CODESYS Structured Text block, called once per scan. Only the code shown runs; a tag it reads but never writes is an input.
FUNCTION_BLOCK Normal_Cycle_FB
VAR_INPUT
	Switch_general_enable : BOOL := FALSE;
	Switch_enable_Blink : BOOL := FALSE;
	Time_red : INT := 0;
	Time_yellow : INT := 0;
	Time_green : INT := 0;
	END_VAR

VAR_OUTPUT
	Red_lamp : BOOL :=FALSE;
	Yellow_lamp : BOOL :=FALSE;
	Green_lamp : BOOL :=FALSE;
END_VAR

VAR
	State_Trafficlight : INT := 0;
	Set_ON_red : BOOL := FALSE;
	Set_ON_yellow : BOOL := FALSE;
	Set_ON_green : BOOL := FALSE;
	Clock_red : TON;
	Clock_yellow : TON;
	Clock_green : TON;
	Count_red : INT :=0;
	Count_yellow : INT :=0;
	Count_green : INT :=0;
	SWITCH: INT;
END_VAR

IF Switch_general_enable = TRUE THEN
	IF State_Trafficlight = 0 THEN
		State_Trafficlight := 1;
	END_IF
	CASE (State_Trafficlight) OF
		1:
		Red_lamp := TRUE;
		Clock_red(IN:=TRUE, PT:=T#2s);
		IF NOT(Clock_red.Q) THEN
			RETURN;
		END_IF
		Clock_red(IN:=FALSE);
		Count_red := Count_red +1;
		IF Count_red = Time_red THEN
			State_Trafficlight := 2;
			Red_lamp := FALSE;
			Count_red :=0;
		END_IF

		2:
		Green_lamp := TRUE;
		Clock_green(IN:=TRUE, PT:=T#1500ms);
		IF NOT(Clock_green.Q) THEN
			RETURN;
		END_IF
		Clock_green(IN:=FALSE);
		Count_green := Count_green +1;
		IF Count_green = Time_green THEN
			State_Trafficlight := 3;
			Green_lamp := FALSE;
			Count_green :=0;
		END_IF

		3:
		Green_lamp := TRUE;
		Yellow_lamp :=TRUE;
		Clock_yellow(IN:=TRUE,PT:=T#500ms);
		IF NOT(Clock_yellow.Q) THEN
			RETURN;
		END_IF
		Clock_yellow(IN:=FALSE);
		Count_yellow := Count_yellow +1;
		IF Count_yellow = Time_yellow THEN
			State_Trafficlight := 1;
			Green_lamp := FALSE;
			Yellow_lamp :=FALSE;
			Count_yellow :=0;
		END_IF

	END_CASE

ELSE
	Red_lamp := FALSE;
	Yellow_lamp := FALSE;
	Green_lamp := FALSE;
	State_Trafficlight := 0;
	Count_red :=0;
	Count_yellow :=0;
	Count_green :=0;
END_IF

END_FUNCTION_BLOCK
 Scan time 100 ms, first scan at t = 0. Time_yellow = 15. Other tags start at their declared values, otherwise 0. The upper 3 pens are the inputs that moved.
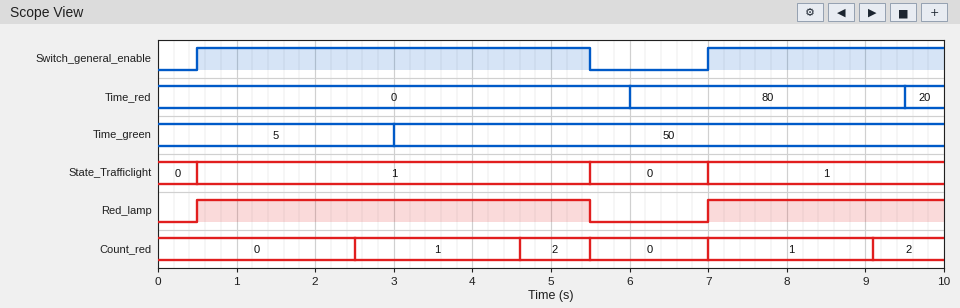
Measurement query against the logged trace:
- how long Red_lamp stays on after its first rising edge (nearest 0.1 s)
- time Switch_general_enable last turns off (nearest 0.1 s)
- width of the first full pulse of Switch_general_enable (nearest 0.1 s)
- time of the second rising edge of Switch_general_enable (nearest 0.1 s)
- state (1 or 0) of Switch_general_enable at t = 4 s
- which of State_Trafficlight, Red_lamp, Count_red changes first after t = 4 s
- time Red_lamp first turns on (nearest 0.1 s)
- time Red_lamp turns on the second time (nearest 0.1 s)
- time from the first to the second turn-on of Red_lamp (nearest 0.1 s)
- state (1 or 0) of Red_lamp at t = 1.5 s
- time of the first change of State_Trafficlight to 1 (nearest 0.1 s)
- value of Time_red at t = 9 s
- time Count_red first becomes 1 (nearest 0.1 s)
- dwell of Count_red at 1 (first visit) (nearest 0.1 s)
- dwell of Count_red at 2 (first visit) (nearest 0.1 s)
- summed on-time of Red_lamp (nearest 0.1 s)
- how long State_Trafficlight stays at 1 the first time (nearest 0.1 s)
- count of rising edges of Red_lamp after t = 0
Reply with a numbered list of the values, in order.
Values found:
1. 5.0 s
2. 5.5 s
3. 5.0 s
4. 7.0 s
5. 1
6. Count_red
7. 0.5 s
8. 7.0 s
9. 6.5 s
10. 1
11. 0.5 s
12. 80
13. 2.5 s
14. 2.1 s
15. 0.9 s
16. 8.0 s
17. 5.0 s
18. 2
